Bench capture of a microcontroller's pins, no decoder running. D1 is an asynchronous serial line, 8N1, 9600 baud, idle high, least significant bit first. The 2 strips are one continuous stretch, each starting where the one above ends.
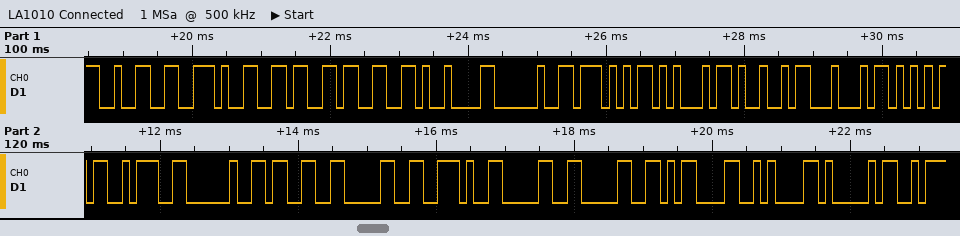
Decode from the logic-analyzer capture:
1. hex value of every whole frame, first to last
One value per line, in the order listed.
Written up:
0x32 0x2E 0x36 0x33 0x09 0x20 0x57 0x45 0x49 0x44 0x55 0x3A 0x20 0x33 0x30 0x2E 0x30 0x30 0x0D 0x0A 0x41
